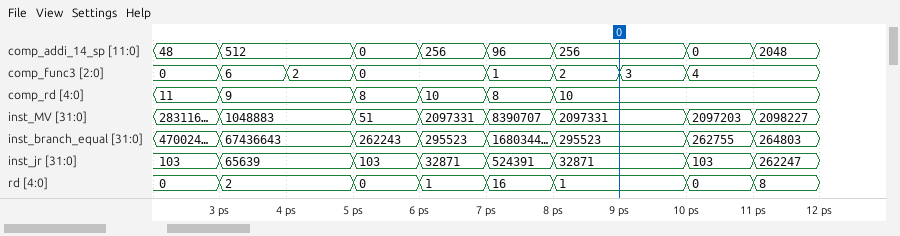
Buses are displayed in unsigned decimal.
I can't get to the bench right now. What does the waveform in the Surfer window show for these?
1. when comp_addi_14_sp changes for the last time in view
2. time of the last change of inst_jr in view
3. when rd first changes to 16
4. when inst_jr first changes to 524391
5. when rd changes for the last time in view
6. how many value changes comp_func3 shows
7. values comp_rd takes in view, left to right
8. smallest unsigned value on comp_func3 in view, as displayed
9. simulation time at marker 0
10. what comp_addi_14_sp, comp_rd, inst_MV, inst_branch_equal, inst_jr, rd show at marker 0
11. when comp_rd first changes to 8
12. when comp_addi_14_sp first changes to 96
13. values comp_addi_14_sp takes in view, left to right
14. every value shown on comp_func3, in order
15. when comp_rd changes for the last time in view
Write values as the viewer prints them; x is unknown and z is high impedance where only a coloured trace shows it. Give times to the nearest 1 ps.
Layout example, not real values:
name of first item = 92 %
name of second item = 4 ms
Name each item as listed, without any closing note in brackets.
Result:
when comp_addi_14_sp changes for the last time in view = 11 ps
time of the last change of inst_jr in view = 11 ps
when rd first changes to 16 = 7 ps
when inst_jr first changes to 524391 = 7 ps
when rd changes for the last time in view = 11 ps
how many value changes comp_func3 shows = 7
values comp_rd takes in view, left to right = 11, 9, 8, 10, 8, 10
smallest unsigned value on comp_func3 in view, as displayed = 0
simulation time at marker 0 = 9 ps
what comp_addi_14_sp, comp_rd, inst_MV, inst_branch_equal, inst_jr, rd show at marker 0 = comp_addi_14_sp=256, comp_rd=10, inst_MV=2097331, inst_branch_equal=295523, inst_jr=32871, rd=1
when comp_rd first changes to 8 = 5 ps
when comp_addi_14_sp first changes to 96 = 7 ps
values comp_addi_14_sp takes in view, left to right = 48, 512, 0, 256, 96, 256, 0, 2048
every value shown on comp_func3, in order = 0, 6, 2, 0, 1, 2, 3, 4
when comp_rd changes for the last time in view = 8 ps
